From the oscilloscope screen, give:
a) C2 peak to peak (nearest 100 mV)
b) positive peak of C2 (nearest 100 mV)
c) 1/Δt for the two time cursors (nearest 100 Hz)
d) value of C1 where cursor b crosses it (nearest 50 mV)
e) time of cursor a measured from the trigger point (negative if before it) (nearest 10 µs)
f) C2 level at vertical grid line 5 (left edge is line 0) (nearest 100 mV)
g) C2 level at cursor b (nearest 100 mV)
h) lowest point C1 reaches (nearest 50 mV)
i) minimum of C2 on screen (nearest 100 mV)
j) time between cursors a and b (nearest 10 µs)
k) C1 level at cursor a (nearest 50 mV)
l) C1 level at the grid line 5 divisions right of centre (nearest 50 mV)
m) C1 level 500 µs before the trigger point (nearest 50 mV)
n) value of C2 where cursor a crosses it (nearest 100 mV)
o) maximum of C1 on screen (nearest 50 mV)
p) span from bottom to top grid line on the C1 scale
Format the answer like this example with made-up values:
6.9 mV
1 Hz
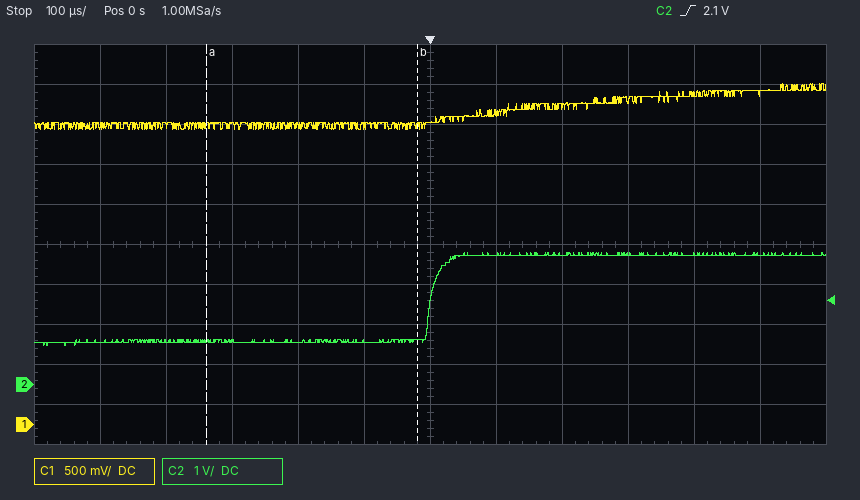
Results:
2.3 V
3.3 V
3.1 kHz
3.75 V
-340 µs
1.1 V
1.1 V
3.70 V
1.0 V
320 µs
3.75 V
4.15 V
3.75 V
1.1 V
4.25 V
5 V
